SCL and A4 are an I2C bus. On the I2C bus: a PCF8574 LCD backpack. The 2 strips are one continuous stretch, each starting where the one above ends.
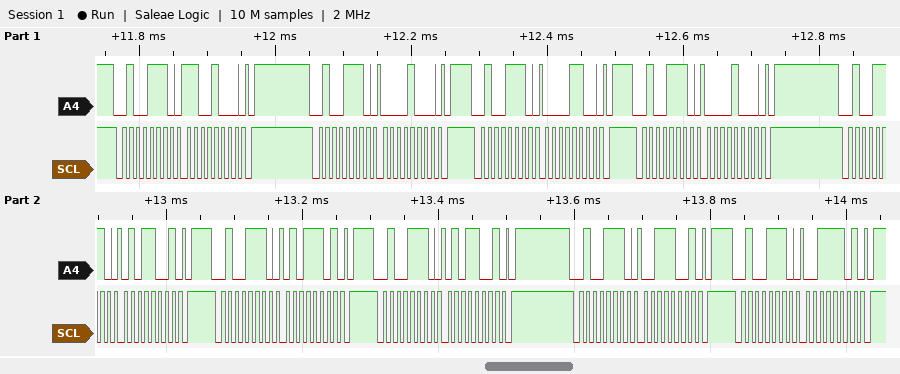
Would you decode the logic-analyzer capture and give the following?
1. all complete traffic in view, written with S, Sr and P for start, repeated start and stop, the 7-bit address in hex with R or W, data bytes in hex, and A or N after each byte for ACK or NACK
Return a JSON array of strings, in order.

["S 27W A C8 A P S 27W A 08 A P S 27W A 0C A P S 27W A 08 A P S 27W A 59 A P S 27W A 5D A P S 27W A 59 A P S 27W A 39 A P S 27W A 3D A P"]
